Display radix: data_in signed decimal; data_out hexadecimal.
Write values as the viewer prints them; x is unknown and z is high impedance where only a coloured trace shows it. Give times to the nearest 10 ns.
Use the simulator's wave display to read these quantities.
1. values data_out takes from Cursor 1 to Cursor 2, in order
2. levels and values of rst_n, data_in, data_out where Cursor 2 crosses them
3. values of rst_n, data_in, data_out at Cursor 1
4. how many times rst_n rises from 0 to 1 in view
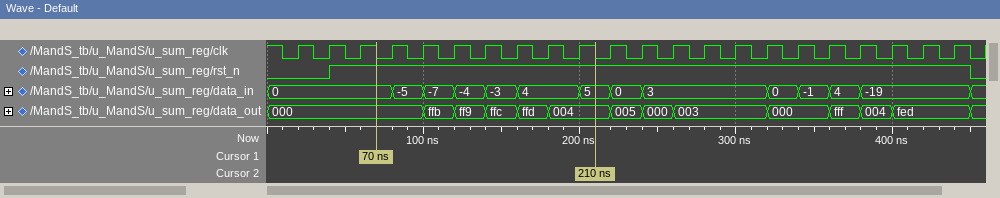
000, ffb, ff9, ffc, ffd, 004
rst_n=1, data_in=5, data_out=004
rst_n=1, data_in=0, data_out=000
1
